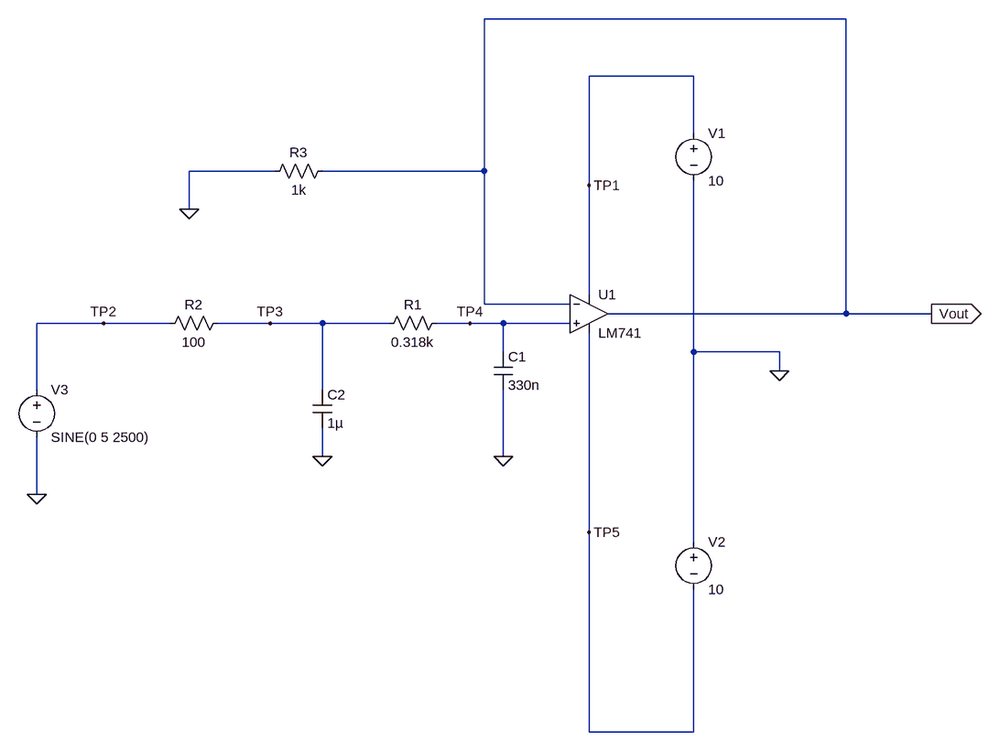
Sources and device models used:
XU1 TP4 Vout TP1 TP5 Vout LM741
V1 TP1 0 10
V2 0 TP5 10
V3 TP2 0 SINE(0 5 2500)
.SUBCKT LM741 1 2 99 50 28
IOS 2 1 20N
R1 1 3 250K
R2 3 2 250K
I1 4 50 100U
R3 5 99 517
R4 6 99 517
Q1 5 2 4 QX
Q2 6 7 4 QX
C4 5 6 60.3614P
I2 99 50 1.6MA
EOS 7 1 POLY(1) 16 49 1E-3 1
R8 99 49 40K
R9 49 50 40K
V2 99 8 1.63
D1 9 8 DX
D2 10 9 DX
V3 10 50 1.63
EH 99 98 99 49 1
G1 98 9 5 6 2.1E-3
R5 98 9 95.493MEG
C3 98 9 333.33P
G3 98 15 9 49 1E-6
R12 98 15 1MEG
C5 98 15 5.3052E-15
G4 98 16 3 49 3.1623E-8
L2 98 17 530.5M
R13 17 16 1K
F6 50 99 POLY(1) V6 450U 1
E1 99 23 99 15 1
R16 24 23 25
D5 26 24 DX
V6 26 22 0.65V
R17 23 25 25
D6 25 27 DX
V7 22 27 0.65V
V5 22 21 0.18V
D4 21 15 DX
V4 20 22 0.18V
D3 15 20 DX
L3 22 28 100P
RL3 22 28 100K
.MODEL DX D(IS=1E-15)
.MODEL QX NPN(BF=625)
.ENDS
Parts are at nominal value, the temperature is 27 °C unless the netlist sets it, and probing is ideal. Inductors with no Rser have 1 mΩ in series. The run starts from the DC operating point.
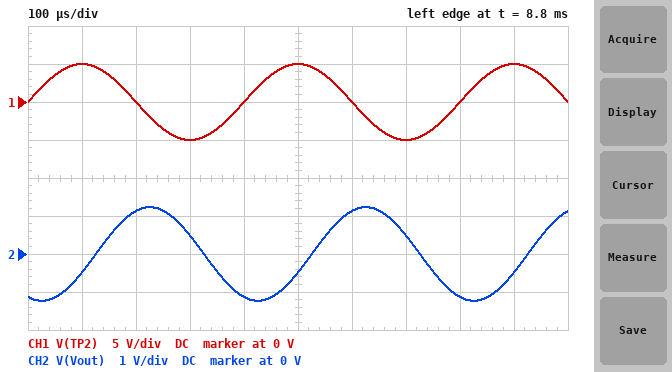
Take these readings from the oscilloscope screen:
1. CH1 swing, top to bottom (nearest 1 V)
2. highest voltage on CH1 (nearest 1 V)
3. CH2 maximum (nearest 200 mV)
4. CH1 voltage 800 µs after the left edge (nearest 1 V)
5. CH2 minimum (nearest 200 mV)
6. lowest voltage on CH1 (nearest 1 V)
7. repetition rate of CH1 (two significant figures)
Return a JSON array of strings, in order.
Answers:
["10 V", "5 V", "1.2 V", "0 V", "-1.2 V", "-5 V", "2.5 kHz"]
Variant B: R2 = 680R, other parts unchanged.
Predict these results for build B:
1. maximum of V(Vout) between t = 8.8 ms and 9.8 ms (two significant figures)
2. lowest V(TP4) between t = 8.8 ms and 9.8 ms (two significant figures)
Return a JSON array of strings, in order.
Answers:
["220 mV", "-220 mV"]
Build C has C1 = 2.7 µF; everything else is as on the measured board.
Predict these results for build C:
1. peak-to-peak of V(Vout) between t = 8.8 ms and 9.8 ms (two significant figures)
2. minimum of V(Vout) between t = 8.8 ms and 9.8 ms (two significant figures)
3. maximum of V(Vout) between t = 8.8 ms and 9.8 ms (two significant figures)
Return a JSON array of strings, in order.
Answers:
["360 mV", "-180 mV", "180 mV"]
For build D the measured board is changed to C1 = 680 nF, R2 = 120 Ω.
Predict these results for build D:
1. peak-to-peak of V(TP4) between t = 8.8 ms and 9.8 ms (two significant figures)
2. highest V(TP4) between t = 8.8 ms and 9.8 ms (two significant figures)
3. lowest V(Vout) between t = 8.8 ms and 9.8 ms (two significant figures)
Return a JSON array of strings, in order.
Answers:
["1.2 V", "590 mV", "-590 mV"]
